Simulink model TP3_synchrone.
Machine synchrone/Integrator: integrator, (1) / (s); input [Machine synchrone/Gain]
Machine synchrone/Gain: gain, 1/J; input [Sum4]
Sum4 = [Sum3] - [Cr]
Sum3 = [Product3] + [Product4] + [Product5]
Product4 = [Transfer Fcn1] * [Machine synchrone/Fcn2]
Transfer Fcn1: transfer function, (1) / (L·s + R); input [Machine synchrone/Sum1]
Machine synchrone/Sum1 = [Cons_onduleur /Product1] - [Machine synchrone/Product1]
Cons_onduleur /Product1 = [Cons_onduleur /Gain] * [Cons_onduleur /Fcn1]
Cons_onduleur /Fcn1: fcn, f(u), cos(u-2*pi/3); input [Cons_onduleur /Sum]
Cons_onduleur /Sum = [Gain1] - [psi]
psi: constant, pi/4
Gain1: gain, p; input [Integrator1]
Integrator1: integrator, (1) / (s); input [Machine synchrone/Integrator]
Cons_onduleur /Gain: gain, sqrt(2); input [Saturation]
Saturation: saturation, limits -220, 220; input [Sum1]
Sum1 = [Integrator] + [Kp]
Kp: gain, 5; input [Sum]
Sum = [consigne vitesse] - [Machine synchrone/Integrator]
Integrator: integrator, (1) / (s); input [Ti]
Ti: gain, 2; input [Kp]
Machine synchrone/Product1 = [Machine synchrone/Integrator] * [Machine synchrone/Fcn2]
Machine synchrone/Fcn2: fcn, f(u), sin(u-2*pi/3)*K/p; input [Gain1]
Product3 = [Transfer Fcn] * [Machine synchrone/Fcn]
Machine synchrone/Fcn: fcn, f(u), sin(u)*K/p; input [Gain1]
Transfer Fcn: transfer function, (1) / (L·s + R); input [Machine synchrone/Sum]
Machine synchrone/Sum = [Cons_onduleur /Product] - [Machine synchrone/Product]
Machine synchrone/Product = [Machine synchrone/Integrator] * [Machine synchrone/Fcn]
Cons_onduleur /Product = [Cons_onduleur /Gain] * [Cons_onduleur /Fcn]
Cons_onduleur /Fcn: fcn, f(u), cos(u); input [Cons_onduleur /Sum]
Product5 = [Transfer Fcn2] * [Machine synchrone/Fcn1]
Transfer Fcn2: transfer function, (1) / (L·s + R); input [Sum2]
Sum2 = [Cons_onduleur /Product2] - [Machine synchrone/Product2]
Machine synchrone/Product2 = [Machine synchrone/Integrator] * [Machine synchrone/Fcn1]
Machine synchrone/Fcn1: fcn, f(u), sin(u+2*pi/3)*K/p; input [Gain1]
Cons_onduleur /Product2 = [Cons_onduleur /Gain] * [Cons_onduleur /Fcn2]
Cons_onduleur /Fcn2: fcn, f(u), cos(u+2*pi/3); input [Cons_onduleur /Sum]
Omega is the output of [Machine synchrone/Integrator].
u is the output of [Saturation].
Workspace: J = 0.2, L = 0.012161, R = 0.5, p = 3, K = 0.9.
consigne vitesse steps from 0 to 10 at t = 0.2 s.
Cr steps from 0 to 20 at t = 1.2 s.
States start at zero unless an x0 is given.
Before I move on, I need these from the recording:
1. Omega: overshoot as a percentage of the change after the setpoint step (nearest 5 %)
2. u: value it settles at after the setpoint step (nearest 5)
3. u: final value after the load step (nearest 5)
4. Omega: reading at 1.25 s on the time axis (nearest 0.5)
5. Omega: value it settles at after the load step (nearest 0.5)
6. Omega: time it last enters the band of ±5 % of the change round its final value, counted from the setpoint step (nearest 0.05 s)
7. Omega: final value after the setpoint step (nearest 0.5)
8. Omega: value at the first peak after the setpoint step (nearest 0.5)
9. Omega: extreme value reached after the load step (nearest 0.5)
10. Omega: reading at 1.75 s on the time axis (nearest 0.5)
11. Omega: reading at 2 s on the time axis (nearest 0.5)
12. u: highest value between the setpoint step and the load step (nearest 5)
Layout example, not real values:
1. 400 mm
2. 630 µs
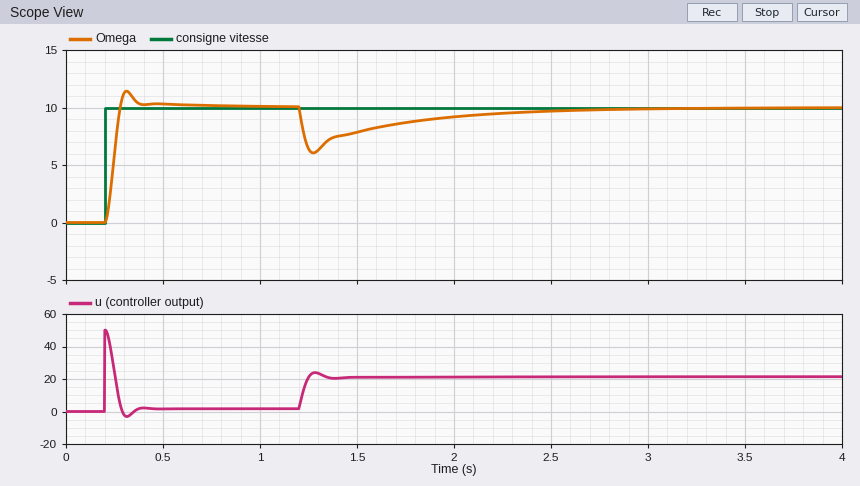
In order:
1. 15 %
2. 0
3. 20
4. 6.5
5. 10.0
6. 0.15 s
7. 10.0
8. 11.5
9. 6.0
10. 8.5
11. 9.0
12. 50
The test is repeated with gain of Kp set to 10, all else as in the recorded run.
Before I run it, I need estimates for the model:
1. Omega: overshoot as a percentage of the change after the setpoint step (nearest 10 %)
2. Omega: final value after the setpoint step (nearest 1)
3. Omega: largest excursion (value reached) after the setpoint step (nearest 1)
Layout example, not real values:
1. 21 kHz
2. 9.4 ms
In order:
1. 30 %
2. 10
3. 13
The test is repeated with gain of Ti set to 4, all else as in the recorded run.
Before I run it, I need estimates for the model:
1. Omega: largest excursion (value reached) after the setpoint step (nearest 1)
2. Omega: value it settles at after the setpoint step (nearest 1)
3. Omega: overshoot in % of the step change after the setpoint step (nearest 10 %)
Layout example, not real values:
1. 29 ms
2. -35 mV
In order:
1. 12
2. 10
3. 20 %
